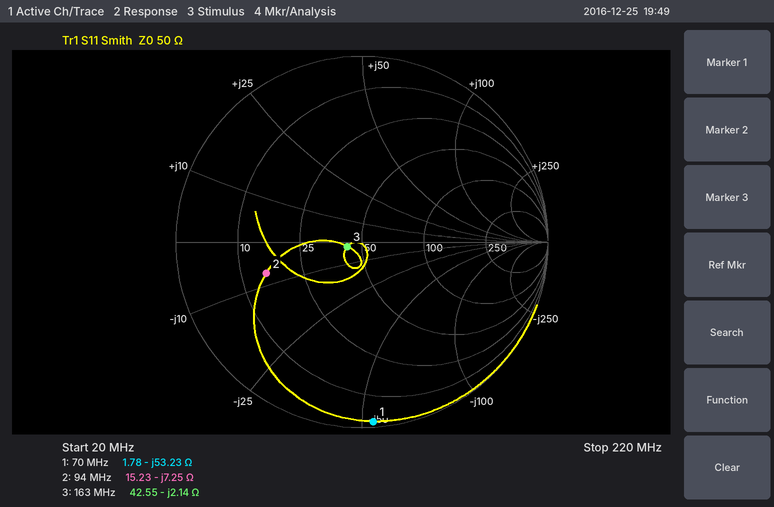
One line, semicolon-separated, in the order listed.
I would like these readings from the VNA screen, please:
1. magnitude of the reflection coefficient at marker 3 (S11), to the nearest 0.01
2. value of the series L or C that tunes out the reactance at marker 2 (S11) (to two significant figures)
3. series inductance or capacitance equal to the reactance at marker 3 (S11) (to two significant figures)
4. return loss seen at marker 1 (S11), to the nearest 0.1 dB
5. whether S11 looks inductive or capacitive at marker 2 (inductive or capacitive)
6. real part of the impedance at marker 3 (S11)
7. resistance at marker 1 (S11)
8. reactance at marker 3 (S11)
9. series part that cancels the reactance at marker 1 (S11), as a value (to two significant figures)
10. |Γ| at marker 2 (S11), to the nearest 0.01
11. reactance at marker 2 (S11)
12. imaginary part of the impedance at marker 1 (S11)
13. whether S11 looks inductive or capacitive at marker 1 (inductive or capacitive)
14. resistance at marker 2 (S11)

0.08; 12 nH; 460 pF; 0.3 dB; capacitive; 42.55 Ω; 1.78 Ω; -2.14 Ω; 120 nH; 0.54; -7.25 Ω; -53.23 Ω; capacitive; 15.23 Ω
